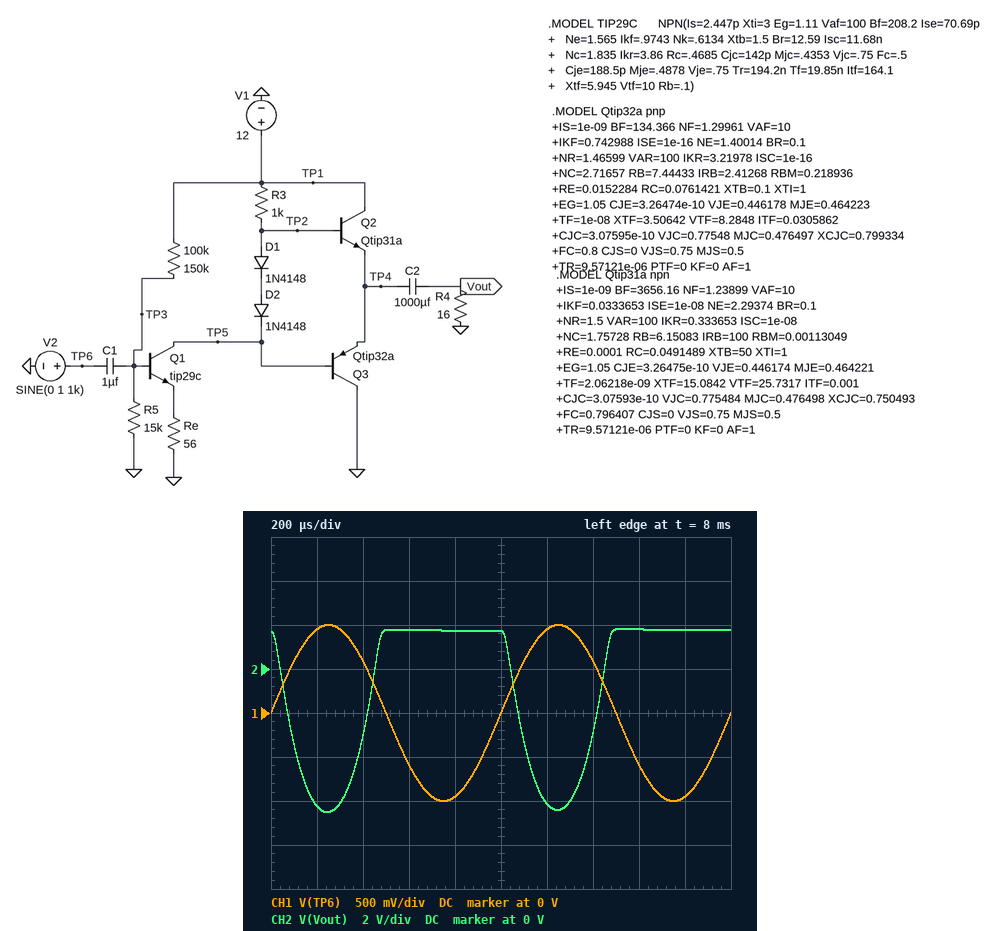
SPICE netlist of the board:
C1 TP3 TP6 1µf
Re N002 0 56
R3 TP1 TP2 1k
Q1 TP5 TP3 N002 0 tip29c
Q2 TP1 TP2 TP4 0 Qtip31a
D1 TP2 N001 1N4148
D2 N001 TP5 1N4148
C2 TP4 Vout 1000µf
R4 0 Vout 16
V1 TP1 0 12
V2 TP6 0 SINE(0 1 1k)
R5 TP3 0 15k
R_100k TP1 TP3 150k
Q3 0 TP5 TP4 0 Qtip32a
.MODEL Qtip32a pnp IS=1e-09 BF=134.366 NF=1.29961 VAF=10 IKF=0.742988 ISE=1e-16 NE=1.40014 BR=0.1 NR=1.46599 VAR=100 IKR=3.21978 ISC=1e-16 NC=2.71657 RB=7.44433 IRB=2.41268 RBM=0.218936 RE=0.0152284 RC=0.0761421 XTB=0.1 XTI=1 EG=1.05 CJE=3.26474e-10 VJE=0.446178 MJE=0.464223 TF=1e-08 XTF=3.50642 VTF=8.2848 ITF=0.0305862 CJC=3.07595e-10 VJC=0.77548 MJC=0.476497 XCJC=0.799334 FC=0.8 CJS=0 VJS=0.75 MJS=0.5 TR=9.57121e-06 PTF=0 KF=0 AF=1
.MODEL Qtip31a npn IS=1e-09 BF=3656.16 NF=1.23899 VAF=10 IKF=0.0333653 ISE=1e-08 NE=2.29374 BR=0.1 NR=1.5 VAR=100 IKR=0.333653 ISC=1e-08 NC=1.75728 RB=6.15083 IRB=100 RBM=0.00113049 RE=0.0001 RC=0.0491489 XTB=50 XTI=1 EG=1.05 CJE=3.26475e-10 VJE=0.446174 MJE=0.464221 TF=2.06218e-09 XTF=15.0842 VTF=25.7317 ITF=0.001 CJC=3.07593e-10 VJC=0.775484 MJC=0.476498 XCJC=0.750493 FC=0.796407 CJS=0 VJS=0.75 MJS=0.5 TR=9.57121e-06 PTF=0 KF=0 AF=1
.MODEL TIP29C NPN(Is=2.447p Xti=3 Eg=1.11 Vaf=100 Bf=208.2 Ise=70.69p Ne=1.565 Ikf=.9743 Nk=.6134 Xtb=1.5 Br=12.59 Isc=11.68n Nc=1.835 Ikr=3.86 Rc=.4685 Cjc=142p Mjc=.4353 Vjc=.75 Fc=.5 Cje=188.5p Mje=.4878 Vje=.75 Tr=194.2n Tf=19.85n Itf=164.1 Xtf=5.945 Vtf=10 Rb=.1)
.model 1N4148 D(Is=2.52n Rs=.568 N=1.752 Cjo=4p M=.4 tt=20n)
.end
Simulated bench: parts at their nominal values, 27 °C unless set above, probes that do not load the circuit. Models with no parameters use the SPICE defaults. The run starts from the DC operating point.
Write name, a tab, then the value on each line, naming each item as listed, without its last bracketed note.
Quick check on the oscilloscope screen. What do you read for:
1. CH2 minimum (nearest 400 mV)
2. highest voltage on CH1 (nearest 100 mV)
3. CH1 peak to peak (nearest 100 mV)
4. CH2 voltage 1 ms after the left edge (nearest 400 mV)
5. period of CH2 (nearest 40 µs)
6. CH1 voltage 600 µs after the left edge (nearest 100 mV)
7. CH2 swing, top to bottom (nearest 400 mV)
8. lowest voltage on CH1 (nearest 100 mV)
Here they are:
CH2 minimum	-6.4 V
highest voltage on CH1	1.0 V
CH1 peak to peak	2.0 V
CH2 voltage 1 ms after the left edge	1.6 V
period of CH2	1.00 ms
CH1 voltage 600 µs after the left edge	-600 mV
CH2 swing, top to bottom	8.4 V
lowest voltage on CH1	-1.0 V
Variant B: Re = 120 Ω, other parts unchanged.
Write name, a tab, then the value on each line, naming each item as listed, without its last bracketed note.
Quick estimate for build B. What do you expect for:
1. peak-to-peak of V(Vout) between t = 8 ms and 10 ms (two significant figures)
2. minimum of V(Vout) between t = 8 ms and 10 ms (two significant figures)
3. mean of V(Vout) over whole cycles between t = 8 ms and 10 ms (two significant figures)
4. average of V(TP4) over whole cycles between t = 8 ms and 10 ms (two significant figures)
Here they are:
peak-to-peak of V(Vout) between t = 8 ms and 10 ms	5.5 V
minimum of V(Vout) between t = 8 ms and 10 ms	-4.2 V
mean of V(Vout) over whole cycles between t = 8 ms and 10 ms	-540 mV
average of V(TP4) over whole cycles between t = 8 ms and 10 ms	9.1 V
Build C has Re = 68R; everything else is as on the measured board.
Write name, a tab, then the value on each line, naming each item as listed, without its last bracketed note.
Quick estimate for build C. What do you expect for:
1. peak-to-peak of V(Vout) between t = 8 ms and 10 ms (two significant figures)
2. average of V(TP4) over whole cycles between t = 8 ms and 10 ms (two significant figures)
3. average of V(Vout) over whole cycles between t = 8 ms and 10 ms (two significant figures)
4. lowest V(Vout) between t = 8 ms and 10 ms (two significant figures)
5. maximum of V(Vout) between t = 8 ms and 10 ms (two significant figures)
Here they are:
peak-to-peak of V(Vout) between t = 8 ms and 10 ms	7.6 V
average of V(TP4) over whole cycles between t = 8 ms and 10 ms	8.4 V
average of V(Vout) over whole cycles between t = 8 ms and 10 ms	-760 mV
lowest V(Vout) between t = 8 ms and 10 ms	-5.9 V
maximum of V(Vout) between t = 8 ms and 10 ms	1.7 V
